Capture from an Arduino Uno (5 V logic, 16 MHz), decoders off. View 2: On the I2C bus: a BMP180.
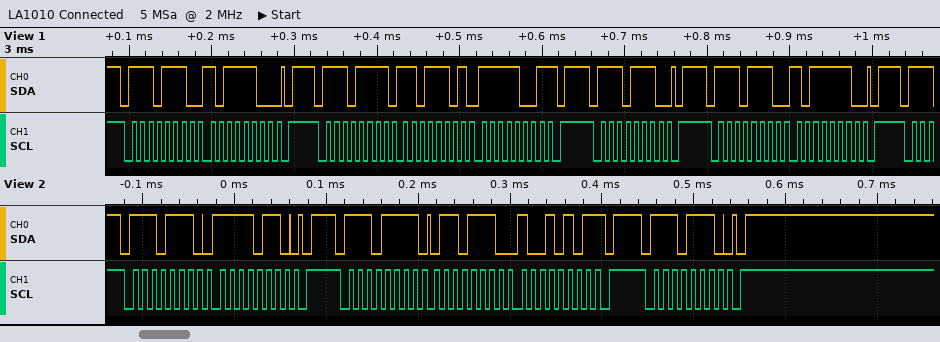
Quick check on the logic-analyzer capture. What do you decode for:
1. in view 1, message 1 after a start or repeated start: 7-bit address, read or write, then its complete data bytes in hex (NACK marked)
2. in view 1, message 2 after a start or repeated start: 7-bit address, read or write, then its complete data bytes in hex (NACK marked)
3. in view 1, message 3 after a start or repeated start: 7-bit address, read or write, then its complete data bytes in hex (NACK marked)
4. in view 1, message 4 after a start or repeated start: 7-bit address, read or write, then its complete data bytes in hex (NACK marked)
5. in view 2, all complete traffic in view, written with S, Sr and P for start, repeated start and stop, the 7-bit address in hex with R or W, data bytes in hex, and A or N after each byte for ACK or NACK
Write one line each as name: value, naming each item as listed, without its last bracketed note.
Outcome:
in view 1, message 1 after a start or repeated start: 7-bit address, read or write, then its complete data bytes in hex: 0x77 write: BC
in view 1, message 2 after a start or repeated start: 7-bit address, read or write, then its complete data bytes in hex: 0x77 read: DD F9 NACK
in view 1, message 3 after a start or repeated start: 7-bit address, read or write, then its complete data bytes in hex: 0x77 write
in view 1, message 4 after a start or repeated start: 7-bit address, read or write, then its complete data bytes in hex: 0x77 write: BE
in view 2, all complete traffic in view, written with S, Sr and P for start, repeated start and stop, the 7-bit address in hex with R or W, data bytes in hex, and A or N after each byte for ACK or NACK: S 77W A F6 A P S 77R A 6E A 95 N P S 77W A P
